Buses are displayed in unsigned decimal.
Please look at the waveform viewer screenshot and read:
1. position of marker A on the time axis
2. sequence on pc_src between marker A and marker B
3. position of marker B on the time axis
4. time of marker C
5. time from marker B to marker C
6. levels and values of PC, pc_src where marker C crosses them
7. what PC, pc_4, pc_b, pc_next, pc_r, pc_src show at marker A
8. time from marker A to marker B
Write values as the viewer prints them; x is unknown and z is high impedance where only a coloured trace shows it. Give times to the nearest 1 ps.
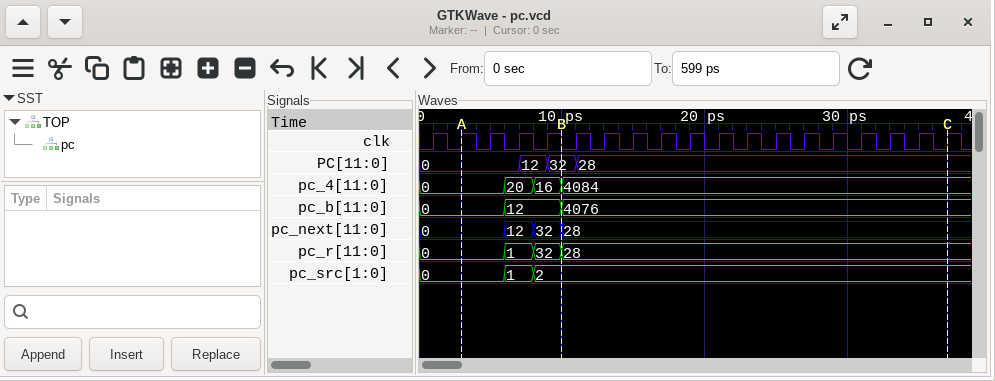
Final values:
3 ps
0, 1, 2
10 ps
37 ps
27 ps
PC=28, pc_src=2
PC=0, pc_4=0, pc_b=0, pc_next=0, pc_r=0, pc_src=0
7 ps
